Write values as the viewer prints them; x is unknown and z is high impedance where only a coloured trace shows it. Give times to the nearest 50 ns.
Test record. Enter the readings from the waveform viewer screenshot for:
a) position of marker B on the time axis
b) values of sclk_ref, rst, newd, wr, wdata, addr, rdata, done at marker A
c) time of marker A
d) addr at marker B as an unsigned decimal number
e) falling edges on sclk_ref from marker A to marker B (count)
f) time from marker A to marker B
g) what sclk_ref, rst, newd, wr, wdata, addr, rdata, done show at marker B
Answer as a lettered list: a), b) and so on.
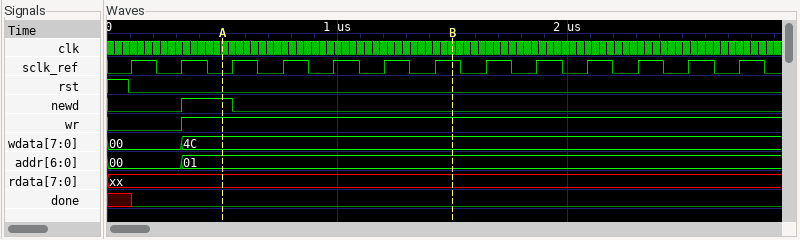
a) 1500 ns
b) sclk_ref=0, rst=0, newd=1, wr=1, wdata=4C, addr=01, rdata=xx, done=0
c) 500 ns
d) 1
e) 4
f) 1000 ns
g) sclk_ref=1, rst=0, newd=0, wr=1, wdata=4C, addr=01, rdata=xx, done=0
